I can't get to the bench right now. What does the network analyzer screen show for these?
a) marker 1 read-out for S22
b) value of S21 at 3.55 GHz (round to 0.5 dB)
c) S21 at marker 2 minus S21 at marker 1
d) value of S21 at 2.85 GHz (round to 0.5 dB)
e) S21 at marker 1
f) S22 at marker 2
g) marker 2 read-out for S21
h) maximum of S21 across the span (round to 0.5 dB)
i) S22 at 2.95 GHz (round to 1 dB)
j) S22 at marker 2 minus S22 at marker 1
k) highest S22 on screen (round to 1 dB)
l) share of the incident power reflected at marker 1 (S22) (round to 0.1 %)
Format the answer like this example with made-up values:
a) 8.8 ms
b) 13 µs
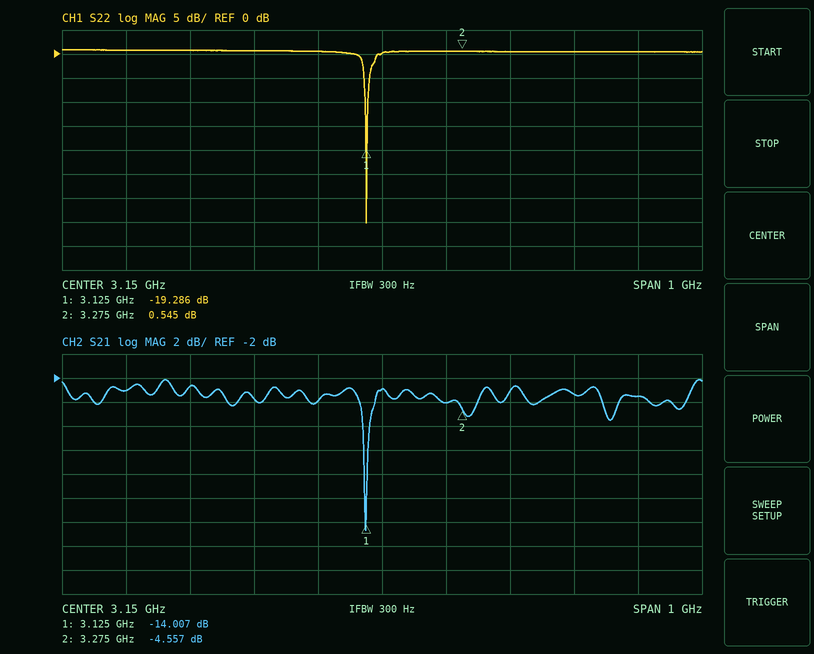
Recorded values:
a) -19.286 dB
b) -3.5 dB
c) 9.450 dB
d) -2.5 dB
e) -14.007 dB
f) 0.545 dB
g) -4.557 dB
h) -2.0 dB
i) 1 dB
j) 19.831 dB
k) 1 dB
l) 1.2 %
